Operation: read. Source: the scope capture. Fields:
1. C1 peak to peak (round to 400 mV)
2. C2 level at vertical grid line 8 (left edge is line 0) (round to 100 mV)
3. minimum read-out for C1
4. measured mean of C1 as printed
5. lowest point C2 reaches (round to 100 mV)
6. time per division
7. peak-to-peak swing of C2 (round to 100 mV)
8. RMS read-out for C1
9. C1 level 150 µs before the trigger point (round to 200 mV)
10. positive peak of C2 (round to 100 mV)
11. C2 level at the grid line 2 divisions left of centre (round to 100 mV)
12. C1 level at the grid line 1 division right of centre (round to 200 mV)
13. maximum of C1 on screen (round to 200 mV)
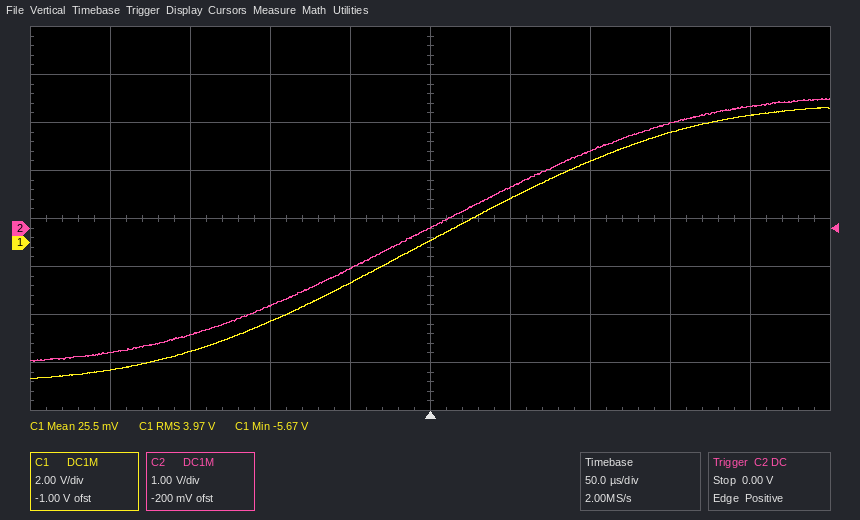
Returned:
11.2 V
2.2 V
-5.67 V
25.5 mV
-2.8 V
50 µs
5.5 V
3.97 V
-4.6 V
2.7 V
-1.6 V
1.8 V
5.6 V
